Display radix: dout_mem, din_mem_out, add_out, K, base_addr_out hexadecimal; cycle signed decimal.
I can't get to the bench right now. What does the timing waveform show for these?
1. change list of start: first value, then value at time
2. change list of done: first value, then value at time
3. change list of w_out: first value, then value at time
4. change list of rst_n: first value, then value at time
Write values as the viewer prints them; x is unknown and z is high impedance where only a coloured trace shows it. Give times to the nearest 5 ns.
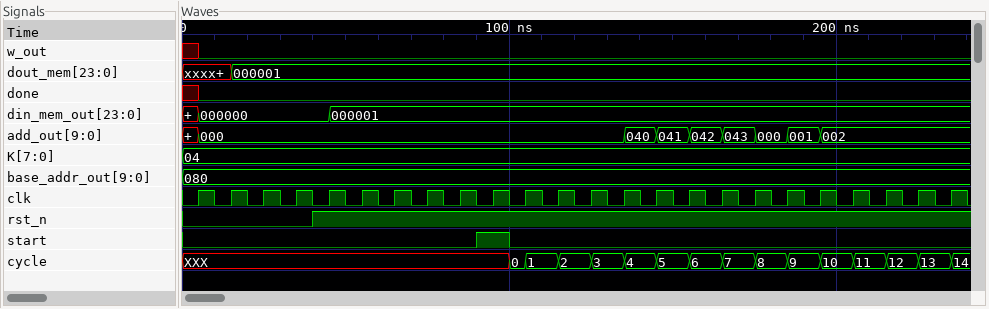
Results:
0, 1 at 90 ns, 0 at 100 ns
x, 0 at 5 ns
x, 0 at 5 ns
0, 1 at 40 ns
